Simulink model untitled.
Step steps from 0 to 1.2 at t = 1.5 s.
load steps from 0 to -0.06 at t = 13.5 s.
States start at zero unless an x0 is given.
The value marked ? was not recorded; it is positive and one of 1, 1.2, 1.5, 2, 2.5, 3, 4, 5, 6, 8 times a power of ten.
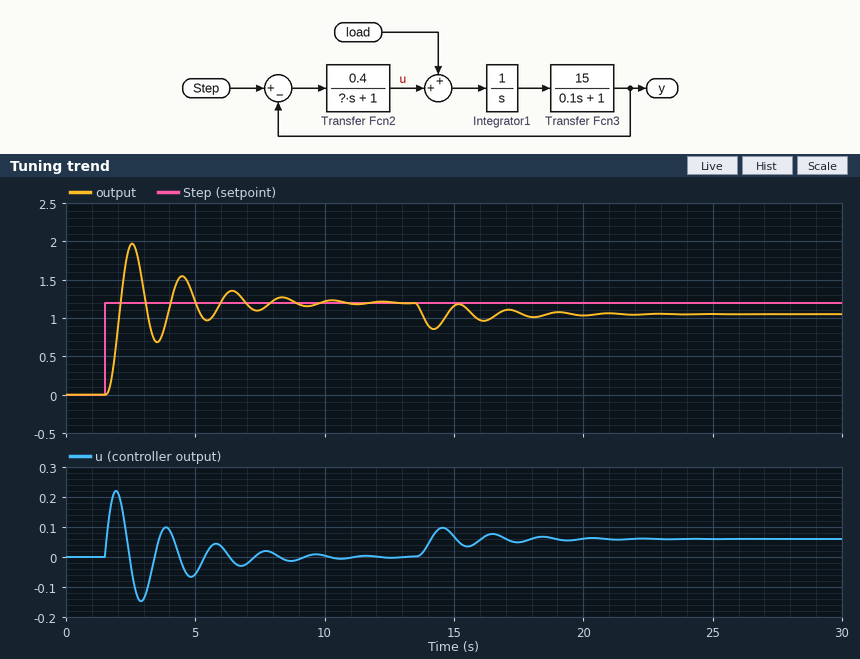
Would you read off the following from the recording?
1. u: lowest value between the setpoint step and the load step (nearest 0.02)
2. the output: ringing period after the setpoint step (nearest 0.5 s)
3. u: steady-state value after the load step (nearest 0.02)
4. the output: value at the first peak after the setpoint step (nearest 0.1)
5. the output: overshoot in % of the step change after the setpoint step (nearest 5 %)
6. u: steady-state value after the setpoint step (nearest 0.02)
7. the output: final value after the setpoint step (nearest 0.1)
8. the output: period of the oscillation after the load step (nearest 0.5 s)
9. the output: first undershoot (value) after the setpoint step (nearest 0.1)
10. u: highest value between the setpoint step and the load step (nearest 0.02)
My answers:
-0.14
2.0 s
0.06
2.0
65 %
0.00
1.2
2.0 s
0.7
0.22
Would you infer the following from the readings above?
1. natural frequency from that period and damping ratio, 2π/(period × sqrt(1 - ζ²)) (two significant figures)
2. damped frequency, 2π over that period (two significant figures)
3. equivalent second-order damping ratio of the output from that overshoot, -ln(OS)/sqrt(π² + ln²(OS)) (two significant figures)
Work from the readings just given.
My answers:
3.2 rad/s
3.1 rad/s
0.14
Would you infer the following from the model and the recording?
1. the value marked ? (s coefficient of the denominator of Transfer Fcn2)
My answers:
0.5
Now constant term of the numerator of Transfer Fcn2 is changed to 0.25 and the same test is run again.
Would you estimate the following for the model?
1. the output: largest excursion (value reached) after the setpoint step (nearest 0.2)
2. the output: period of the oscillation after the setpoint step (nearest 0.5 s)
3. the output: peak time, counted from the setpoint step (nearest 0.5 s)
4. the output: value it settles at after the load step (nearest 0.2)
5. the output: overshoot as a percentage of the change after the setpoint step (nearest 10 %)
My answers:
1.8
2.5 s
1.5 s
1.0
50 %
